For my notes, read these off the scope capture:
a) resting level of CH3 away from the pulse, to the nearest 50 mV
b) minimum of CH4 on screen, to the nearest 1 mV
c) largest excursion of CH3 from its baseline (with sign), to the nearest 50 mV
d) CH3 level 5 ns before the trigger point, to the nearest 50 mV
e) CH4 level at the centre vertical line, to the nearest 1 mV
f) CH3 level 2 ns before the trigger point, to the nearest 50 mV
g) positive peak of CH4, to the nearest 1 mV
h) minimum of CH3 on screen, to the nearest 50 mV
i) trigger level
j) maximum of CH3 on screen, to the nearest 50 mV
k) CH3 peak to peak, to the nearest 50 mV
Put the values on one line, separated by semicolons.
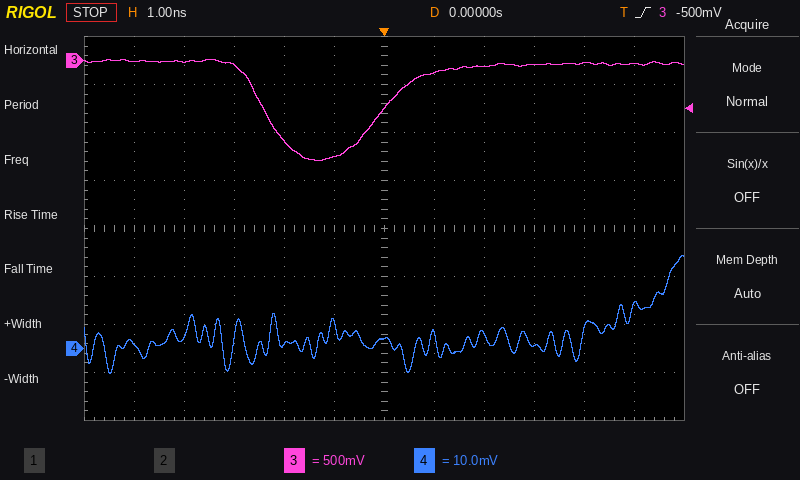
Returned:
-50 mV; -5 mV; -1.00 V; 0 mV; 2 mV; -850 mV; 19 mV; -1.05 V; -500 mV; 0 mV; 1.05 V
